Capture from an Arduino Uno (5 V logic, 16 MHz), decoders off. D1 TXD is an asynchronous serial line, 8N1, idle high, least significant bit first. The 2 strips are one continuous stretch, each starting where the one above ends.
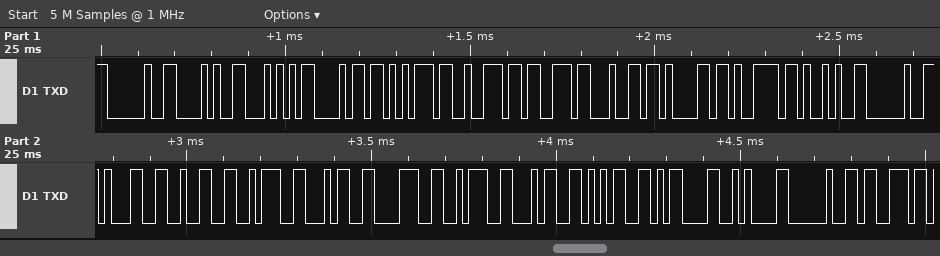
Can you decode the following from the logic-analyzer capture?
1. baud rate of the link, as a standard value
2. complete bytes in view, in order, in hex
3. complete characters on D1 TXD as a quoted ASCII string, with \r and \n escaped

57600 baud
20 28 54 68 75 72 73 64 61 79 29 20 31 32 3A 34 38 3A 34 35 0D 0A 20 73
" (Thursday) 12:48:45\r\n s"
